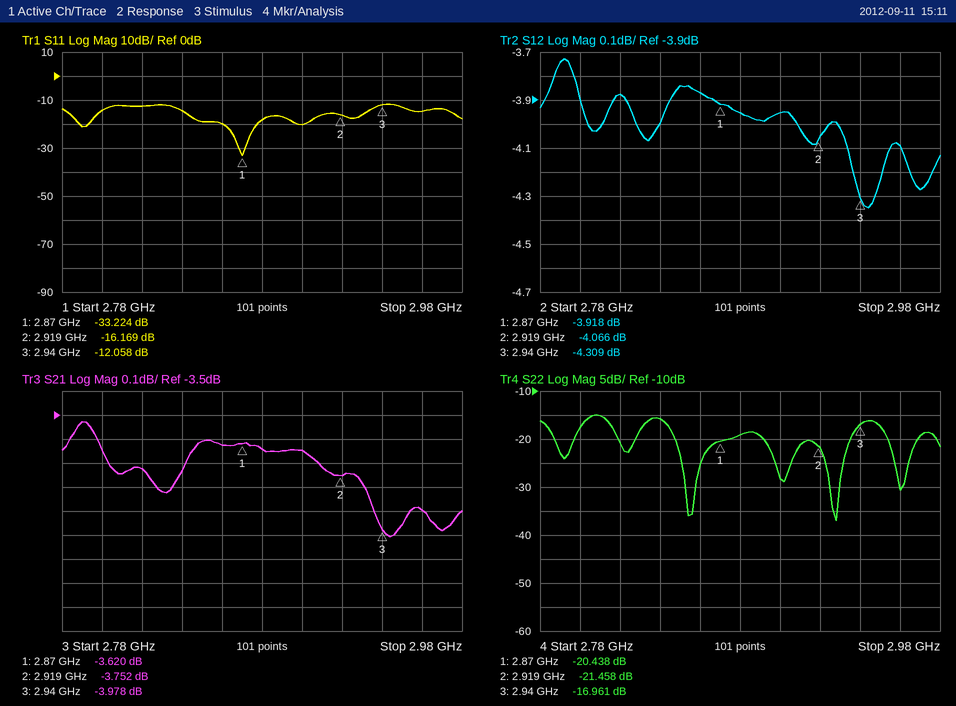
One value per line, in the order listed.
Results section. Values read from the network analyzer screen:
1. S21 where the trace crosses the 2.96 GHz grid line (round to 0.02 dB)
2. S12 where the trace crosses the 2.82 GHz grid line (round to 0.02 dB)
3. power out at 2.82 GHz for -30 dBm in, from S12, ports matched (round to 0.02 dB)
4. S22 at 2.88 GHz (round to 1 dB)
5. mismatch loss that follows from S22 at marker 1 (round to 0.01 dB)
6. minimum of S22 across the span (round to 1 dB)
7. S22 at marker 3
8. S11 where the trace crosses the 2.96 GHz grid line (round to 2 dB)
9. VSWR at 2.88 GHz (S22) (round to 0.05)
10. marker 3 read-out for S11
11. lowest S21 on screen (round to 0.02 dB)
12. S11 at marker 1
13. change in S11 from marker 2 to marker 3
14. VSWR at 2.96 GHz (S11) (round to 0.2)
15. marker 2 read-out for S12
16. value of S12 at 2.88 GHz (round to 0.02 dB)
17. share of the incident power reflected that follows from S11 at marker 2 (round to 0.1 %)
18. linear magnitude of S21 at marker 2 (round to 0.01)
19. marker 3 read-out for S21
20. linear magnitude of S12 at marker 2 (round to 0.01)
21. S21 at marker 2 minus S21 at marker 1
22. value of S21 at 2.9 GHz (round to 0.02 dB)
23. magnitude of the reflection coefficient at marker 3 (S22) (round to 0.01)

-3.90 dB
-3.88 dB
-33.88 dBm
-19 dB
0.04 dB
-37 dB
-16.961 dB
-14 dB
1.25
-12.058 dB
-4.00 dB
-33.224 dB
4.111 dB
1.4
-4.066 dB
-3.96 dB
2.4 %
0.65
-3.978 dB
0.63
-0.132 dB
-3.64 dB
0.14
